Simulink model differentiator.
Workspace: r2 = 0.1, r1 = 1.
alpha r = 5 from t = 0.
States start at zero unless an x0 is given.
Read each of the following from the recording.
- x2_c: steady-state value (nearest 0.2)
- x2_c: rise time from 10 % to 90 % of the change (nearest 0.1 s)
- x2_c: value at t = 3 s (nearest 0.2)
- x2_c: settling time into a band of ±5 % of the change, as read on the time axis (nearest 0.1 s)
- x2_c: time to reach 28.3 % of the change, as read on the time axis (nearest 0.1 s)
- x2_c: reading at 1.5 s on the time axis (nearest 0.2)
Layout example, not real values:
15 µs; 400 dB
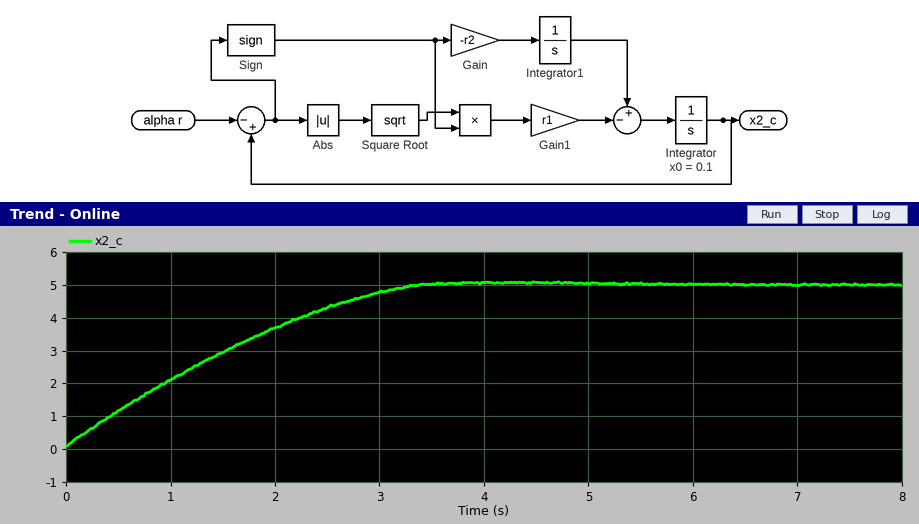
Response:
5.0; 2.5 s; 4.8; 3.0 s; 0.7 s; 3.0
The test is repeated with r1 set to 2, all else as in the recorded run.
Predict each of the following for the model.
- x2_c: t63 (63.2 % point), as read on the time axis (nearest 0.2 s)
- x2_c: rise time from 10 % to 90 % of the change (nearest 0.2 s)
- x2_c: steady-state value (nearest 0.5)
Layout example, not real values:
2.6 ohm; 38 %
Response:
0.8 s; 1.4 s; 5.0
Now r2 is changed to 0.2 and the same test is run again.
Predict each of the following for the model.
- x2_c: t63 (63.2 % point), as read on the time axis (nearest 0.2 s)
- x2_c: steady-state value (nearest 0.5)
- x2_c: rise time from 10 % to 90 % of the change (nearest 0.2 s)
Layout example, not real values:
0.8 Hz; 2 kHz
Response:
1.6 s; 5.0; 2.2 s
